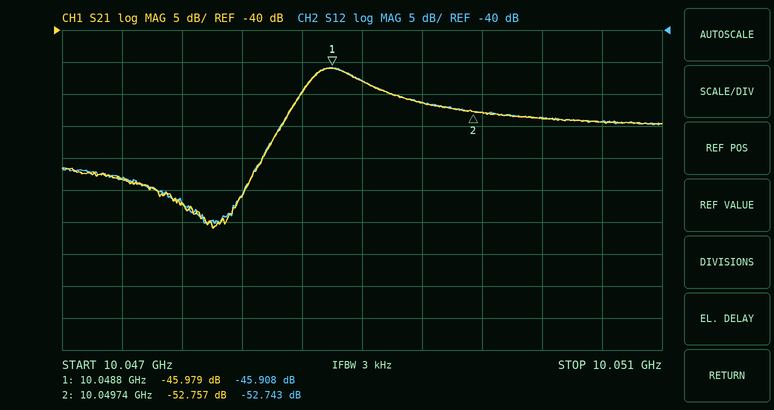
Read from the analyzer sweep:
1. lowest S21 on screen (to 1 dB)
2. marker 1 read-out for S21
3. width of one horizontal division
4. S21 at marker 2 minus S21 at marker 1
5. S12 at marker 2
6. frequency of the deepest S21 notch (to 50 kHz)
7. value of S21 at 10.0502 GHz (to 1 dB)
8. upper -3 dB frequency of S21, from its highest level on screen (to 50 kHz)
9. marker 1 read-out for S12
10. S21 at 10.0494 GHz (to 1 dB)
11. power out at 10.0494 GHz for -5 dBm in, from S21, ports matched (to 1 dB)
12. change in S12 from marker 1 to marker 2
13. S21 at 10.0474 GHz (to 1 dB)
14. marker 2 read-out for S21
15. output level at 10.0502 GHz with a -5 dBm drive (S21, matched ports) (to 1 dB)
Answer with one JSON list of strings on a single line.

["-71 dB", "-45.979 dB", "400 kHz", "-6.778 dB", "-52.743 dB", "10.04800 GHz", "-54 dB", "10.04910 GHz", "-45.908 dB", "-51 dB", "-56 dBm", "-6.835 dB", "-63 dB", "-52.757 dB", "-59 dBm"]
